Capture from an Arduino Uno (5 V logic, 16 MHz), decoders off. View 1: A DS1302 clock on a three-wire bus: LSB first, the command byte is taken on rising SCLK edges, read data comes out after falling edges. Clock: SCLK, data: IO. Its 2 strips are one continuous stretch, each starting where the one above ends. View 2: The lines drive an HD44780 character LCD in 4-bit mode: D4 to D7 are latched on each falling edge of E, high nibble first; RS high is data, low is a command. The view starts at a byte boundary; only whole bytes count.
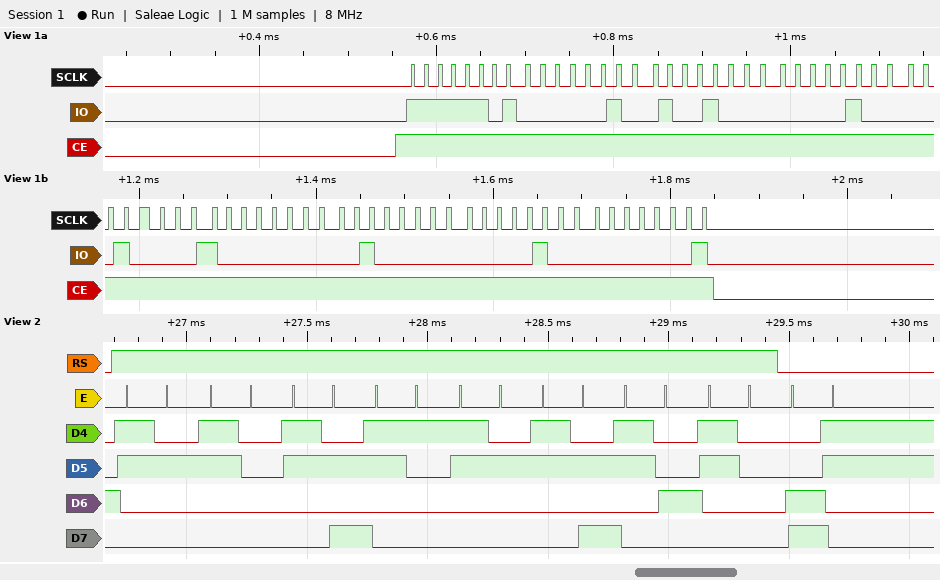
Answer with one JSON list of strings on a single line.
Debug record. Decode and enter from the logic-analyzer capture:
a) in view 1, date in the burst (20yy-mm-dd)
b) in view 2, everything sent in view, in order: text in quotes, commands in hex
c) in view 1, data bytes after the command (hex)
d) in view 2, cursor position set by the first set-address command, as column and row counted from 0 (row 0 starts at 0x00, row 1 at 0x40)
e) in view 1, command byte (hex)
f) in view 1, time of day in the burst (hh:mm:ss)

["2020-01-08", "\"20:12:40\" 0xC3", "40 12 20 08 01 04 20 80", "column 3, row 1", "0xBF", "20:12:40"]
